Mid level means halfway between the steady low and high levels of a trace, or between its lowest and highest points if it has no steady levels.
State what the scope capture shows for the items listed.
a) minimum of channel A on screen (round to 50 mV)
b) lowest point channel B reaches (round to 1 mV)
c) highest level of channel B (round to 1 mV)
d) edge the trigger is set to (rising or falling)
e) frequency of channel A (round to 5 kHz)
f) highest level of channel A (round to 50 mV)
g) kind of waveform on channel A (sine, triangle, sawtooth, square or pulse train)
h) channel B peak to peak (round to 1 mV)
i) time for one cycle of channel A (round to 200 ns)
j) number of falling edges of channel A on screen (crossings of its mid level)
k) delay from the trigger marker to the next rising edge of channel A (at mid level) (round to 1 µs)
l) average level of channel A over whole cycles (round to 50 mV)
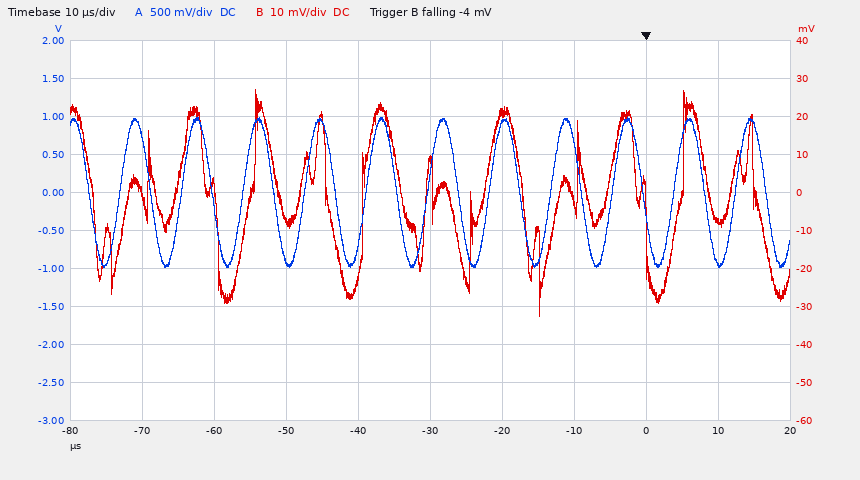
-1.00 V
-33 mV
27 mV
falling
115 kHz
1.00 V
sine
60 mV
8.6 µs
12
4 µs
0 mV
